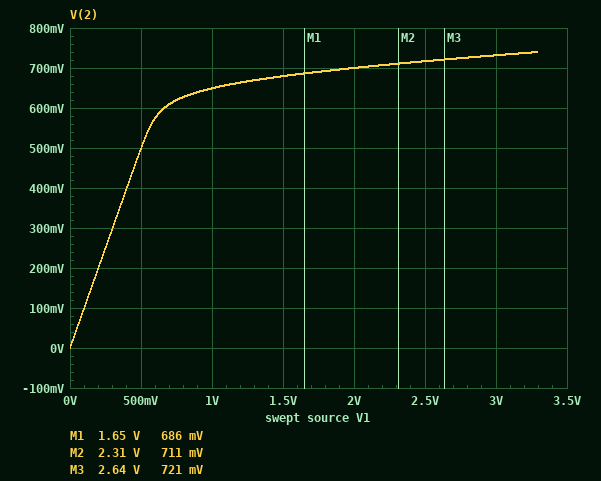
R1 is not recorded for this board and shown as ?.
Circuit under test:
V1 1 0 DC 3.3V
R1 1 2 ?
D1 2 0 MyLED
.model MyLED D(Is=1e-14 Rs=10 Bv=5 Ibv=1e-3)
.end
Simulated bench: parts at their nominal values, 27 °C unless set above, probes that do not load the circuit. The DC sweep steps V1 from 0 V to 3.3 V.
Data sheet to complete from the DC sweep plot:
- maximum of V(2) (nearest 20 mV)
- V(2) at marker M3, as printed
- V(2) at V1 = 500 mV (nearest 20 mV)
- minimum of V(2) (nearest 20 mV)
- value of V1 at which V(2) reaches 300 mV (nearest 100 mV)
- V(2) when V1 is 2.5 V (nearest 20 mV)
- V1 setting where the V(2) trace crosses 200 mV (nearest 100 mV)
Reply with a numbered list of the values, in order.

1. 740 mV
2. 721 mV
3. 500 mV
4. 0 V
5. 300 mV
6. 720 mV
7. 200 mV
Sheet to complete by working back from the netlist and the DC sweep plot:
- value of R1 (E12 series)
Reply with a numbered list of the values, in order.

1. 560 Ω
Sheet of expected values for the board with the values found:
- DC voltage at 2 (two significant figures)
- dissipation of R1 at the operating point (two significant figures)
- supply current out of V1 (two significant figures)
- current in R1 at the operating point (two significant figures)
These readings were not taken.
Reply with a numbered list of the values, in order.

1. 740 mV
2. 12 mW
3. 4.6 mA
4. 4.6 mA
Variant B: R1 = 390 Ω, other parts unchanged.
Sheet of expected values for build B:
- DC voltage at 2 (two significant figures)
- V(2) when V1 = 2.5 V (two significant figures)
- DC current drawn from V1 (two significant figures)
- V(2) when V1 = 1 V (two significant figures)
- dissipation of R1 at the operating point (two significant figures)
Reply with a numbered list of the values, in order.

1. 770 mV
2. 740 mV
3. 6.5 mA
4. 660 mV
5. 16 mW
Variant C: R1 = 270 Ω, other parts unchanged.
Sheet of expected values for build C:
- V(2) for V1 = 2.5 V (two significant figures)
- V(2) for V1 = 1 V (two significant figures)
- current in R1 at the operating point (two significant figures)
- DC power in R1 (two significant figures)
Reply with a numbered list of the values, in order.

1. 770 mV
2. 670 mV
3. 9.2 mA
4. 23 mW
